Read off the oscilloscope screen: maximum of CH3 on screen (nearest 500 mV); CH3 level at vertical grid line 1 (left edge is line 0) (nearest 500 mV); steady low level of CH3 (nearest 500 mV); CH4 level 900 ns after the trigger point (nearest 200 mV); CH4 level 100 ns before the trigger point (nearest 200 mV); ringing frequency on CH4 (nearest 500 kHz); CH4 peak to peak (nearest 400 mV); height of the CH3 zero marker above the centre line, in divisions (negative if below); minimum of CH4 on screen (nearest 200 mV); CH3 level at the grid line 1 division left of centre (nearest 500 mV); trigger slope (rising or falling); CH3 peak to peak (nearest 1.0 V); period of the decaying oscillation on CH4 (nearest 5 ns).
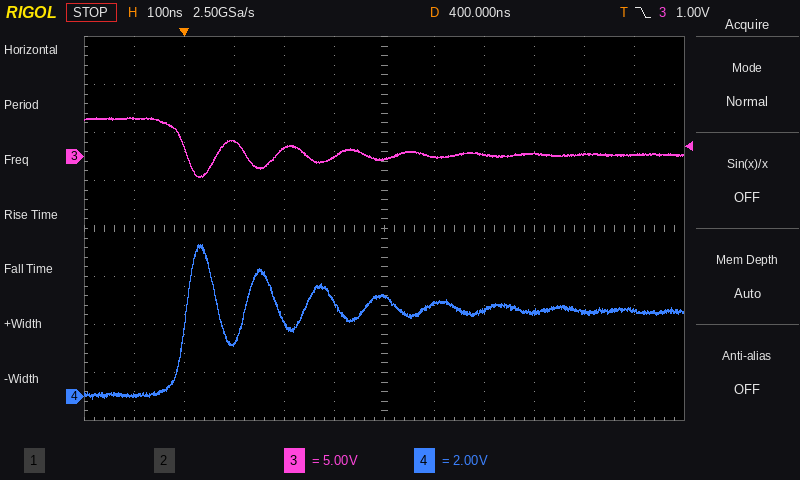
4.0 V
4.0 V
0.0 V
3.6 V
0.0 V
8.5 MHz
6.4 V
+1.5 div
-200 mV
0.0 V
falling
6.0 V
120 ns
